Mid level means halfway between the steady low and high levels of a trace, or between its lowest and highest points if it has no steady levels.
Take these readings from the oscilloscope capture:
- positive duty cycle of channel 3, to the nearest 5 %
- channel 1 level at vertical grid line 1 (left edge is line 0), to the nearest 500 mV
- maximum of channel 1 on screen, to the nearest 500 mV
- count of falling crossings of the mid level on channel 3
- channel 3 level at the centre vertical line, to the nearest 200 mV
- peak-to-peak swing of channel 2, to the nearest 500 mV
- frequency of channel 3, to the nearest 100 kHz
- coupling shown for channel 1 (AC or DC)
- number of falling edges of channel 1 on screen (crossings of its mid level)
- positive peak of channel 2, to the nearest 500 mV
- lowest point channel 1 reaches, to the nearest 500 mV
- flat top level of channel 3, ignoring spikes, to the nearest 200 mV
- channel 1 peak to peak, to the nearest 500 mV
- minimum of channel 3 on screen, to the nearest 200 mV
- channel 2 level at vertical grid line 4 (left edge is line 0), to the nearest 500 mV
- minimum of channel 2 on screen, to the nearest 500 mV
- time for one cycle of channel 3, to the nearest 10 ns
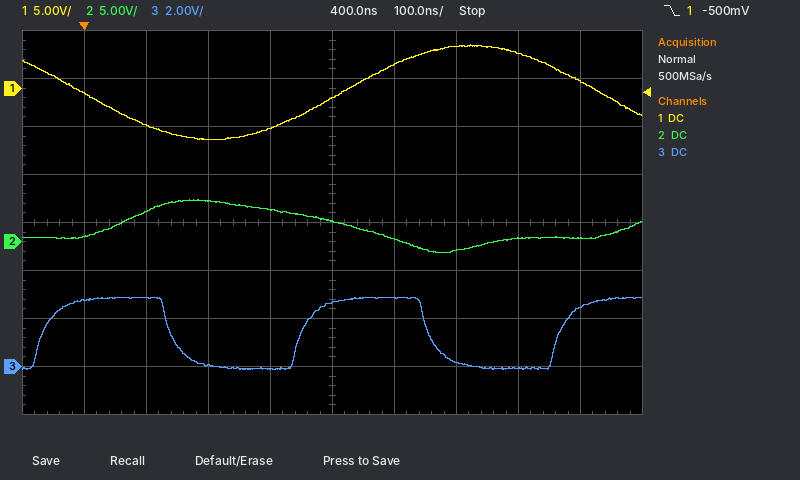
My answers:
50 %
-500 mV
4.5 V
2
2.6 V
5.5 V
2.4 MHz
DC
2
4.5 V
-5.5 V
2.8 V
10.0 V
-200 mV
3.5 V
-1.0 V
420 ns
